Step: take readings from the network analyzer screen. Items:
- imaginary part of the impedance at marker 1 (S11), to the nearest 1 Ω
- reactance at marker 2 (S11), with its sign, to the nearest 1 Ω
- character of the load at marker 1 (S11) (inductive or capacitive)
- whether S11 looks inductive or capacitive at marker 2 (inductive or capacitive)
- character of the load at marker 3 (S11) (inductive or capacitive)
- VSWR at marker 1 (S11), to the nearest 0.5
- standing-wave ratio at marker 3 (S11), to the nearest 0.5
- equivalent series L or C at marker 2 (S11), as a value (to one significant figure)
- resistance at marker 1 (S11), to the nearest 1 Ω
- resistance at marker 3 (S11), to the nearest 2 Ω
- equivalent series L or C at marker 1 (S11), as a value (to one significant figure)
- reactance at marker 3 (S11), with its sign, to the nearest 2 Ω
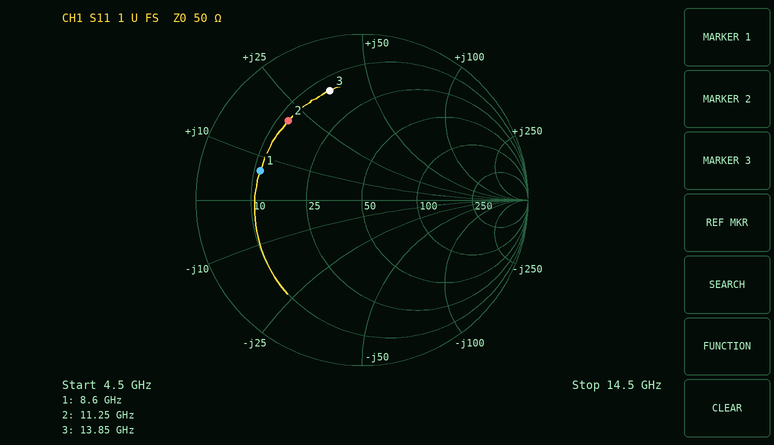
+7 Ω
+21 Ω
inductive
inductive
inductive
4.5
5.5
300 pH
11 Ω
14 Ω
100 pH
+36 Ω
